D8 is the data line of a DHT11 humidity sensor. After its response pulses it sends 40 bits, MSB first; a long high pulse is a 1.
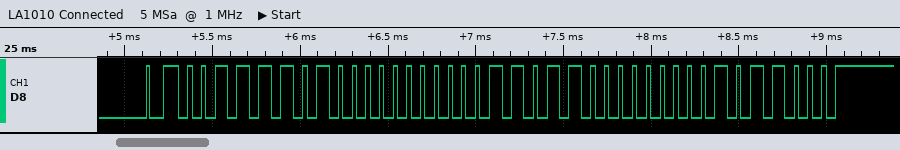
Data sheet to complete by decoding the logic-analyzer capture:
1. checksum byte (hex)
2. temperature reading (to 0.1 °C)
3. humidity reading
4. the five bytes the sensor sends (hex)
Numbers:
0x58
27.0 °C
61 %
3D 00 1B 00 58
